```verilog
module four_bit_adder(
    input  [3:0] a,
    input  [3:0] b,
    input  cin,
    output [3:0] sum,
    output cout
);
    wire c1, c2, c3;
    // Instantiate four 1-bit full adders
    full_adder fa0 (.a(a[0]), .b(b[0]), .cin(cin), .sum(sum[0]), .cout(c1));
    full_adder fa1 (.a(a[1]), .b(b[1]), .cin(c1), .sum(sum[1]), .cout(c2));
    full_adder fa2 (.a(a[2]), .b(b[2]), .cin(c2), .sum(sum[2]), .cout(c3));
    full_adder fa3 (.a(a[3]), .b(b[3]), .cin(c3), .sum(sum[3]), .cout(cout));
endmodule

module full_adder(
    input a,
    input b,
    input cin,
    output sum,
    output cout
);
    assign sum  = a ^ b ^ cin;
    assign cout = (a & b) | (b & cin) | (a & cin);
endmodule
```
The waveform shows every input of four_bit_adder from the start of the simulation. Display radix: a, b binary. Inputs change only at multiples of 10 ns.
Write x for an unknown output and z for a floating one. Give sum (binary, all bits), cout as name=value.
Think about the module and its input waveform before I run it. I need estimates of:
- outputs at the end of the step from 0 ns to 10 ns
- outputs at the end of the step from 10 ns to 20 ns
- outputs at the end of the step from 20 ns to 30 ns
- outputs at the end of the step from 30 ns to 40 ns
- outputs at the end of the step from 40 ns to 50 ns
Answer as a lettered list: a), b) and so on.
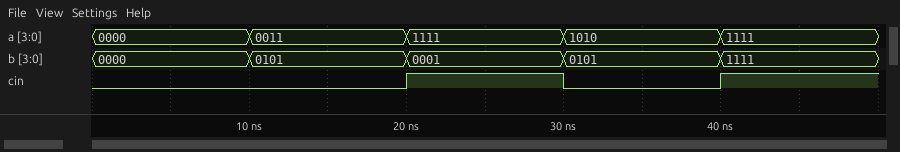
a) sum=0000, cout=0
b) sum=1000, cout=0
c) sum=0001, cout=1
d) sum=1111, cout=0
e) sum=1111, cout=1
